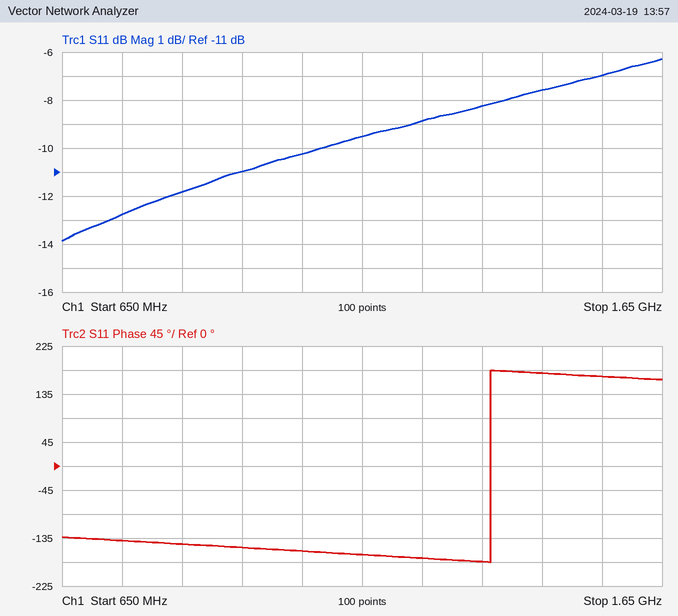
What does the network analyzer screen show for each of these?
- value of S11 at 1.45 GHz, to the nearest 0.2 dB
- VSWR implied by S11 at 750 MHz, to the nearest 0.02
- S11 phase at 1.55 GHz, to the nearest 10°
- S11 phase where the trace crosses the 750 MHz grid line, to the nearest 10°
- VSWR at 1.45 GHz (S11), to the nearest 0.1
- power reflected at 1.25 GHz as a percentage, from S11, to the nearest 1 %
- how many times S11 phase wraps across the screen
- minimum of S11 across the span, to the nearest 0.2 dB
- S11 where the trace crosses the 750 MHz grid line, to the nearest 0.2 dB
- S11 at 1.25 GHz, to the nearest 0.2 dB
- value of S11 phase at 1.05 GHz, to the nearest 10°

-7.6 dB
1.60
170°
-140°
2.4
13 %
1
-13.8 dB
-12.8 dB
-8.8 dB
-160°
